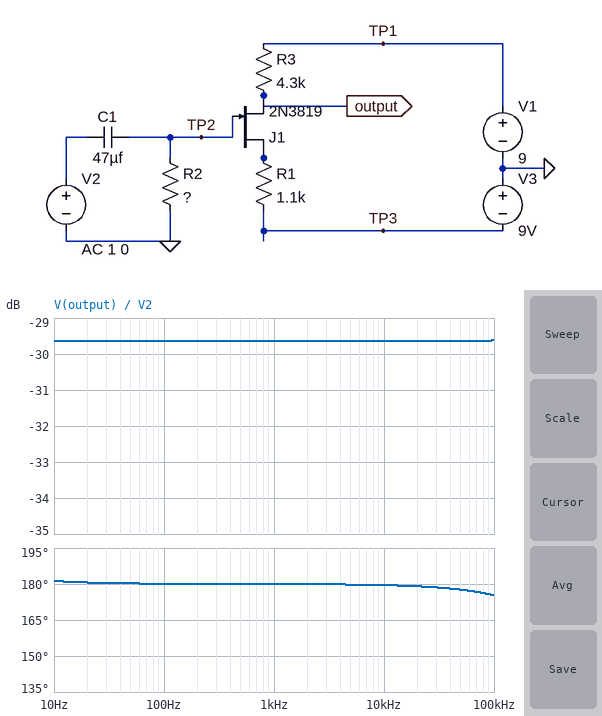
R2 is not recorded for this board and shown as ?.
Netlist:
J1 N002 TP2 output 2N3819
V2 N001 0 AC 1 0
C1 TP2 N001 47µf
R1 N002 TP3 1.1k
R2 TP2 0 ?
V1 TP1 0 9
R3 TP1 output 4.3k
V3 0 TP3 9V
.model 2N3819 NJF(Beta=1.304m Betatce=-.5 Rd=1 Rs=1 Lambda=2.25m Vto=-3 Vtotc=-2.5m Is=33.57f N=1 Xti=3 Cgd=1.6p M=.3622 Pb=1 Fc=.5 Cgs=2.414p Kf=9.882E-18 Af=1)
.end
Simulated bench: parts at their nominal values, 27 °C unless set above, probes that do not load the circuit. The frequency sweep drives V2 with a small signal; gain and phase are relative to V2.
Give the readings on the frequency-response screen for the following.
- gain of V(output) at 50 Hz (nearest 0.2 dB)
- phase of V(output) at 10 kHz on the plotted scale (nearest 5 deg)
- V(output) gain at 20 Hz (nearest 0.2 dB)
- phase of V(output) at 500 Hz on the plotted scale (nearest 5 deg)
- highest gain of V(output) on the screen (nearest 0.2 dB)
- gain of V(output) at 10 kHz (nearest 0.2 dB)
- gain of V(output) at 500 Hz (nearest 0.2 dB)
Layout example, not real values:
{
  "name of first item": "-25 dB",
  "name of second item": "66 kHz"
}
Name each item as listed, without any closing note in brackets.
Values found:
{
  "gain of V(output) at 50 Hz": "-29.6 dB",
  "phase of V(output) at 10 kHz on the plotted scale": "180 deg",
  "V(output) gain at 20 Hz": "-29.6 dB",
  "phase of V(output) at 500 Hz on the plotted scale": "180 deg",
  "highest gain of V(output) on the screen": "-29.6 dB",
  "gain of V(output) at 10 kHz": "-29.6 dB",
  "gain of V(output) at 500 Hz": "-29.6 dB"
}
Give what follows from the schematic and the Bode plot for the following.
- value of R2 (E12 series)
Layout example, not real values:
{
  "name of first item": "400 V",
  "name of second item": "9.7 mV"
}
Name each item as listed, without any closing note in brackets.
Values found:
{
  "value of R2": "2.7 MΩ"
}
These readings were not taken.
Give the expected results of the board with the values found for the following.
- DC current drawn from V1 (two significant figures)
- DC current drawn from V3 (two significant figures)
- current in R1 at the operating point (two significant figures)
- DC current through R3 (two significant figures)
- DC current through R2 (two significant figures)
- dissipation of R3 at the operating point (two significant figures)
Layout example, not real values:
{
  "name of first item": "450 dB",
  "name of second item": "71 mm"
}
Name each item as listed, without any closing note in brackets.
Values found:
{
  "DC current drawn from V1": "3.3 mA",
  "DC current drawn from V3": "3.3 mA",
  "current in R1 at the operating point": "3.3 mA",
  "DC current through R3": "3.3 mA",
  "DC current through R2": "1.8 µA",
  "dissipation of R3 at the operating point": "46 mW"
}
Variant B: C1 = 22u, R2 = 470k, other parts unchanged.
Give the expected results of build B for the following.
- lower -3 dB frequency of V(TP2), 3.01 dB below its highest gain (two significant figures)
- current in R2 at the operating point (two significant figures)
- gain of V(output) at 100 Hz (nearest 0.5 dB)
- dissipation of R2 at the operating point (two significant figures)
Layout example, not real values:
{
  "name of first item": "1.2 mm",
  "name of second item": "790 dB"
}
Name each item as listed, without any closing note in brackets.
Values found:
{
  "lower -3 dB frequency of V(TP2), 3.01 dB below its highest gain": "2.1 Hz",
  "current in R2 at the operating point": "10 µA",
  "gain of V(output) at 100 Hz": "-15.0 dB",
  "dissipation of R2 at the operating point": "51 µW"
}
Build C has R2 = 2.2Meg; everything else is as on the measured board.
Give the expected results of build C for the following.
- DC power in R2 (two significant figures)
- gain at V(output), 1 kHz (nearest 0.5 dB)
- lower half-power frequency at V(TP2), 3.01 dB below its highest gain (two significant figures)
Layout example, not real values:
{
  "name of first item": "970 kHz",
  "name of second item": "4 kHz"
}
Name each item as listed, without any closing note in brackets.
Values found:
{
  "DC power in R2": "11 µW",
  "gain at V(output), 1 kHz": "-34.0 dB",
  "lower half-power frequency at V(TP2), 3.01 dB below its highest gain": "270 mHz"
}
